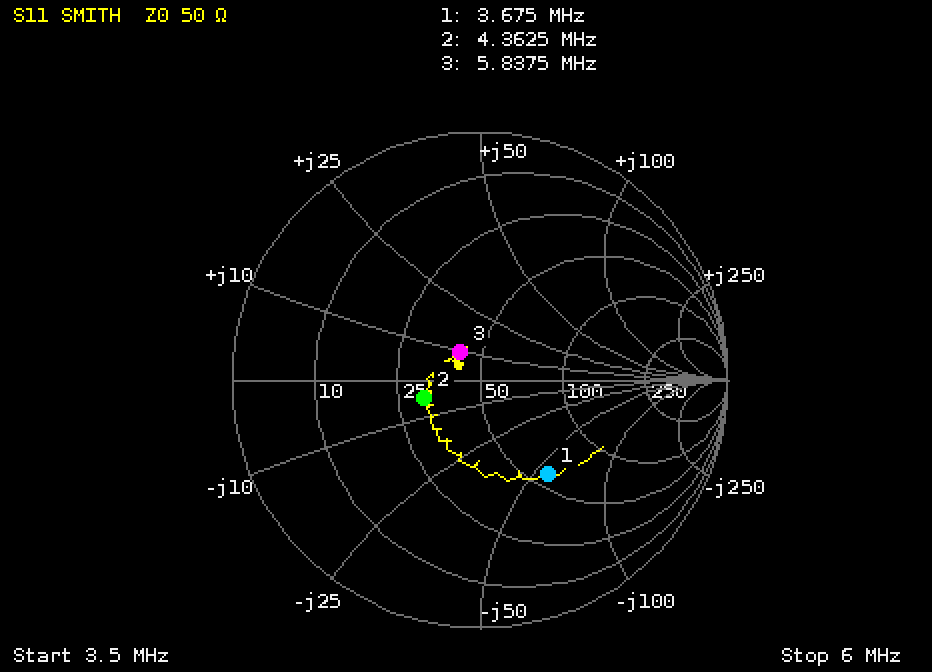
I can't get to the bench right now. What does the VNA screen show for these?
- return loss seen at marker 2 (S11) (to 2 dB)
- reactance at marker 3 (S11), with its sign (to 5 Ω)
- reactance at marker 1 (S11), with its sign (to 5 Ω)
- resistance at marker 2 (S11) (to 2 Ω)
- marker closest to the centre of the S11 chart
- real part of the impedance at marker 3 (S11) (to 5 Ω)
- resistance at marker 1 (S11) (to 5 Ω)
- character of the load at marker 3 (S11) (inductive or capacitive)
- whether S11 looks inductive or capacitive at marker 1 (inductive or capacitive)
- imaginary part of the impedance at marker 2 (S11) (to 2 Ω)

12 dB
+10 Ω
-55 Ω
32 Ω
marker 3
40 Ω
60 Ω
inductive
capacitive
-4 Ω
